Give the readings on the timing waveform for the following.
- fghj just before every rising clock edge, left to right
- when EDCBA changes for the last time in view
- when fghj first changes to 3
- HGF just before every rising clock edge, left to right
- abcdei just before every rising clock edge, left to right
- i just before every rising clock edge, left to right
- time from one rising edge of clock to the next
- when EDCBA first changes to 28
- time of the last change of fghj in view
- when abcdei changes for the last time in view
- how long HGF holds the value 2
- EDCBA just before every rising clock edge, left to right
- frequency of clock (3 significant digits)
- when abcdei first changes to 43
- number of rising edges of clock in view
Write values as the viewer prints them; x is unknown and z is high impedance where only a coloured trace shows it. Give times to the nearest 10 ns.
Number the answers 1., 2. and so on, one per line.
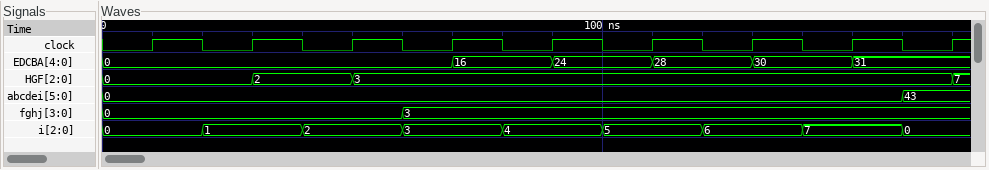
1. 0, 0, 0, 3, 3, 3, 3, 3, 3
2. 150 ns
3. 60 ns
4. 0, 0, 2, 3, 3, 3, 3, 3, 3
5. 0, 0, 0, 0, 0, 0, 0, 0, 43
6. 0, 1, 2, 3, 4, 5, 6, 7, 0
7. 20 ns
8. 110 ns
9. 60 ns
10. 160 ns
11. 20 ns
12. 0, 0, 0, 0, 16, 24, 28, 30, 31
13. 50.0 MHz
14. 160 ns
15. 9
